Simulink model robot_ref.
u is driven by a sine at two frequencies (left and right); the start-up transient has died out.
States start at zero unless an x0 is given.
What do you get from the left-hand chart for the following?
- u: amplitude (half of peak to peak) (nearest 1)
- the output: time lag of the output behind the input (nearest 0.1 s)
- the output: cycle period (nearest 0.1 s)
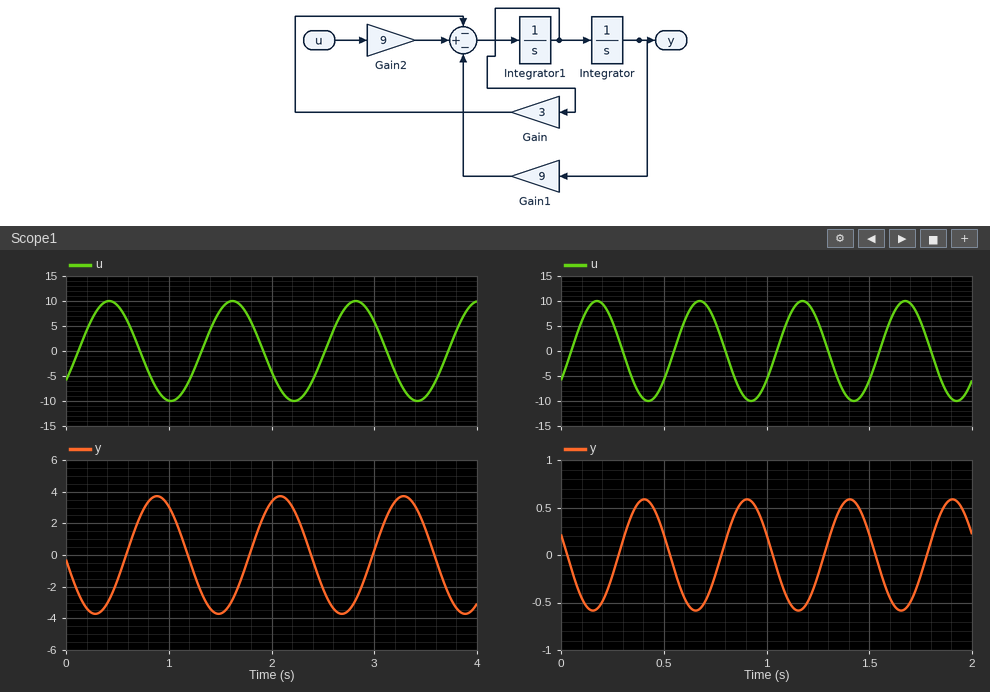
10
0.5 s
1.2 s
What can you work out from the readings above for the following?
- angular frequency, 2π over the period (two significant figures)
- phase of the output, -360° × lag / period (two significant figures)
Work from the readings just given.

5.2 rad/s
-150°
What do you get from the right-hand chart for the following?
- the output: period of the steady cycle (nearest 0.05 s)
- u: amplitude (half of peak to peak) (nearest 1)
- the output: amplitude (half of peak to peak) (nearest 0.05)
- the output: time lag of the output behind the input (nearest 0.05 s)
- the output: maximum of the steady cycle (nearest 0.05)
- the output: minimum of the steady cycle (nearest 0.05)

0.50 s
10
0.60
0.25 s
0.60
-0.60
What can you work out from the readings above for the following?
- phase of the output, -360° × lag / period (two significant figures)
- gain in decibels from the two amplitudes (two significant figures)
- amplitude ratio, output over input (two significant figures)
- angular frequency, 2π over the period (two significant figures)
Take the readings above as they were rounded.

-180°
-24 dB
0.060
13 rad/s
